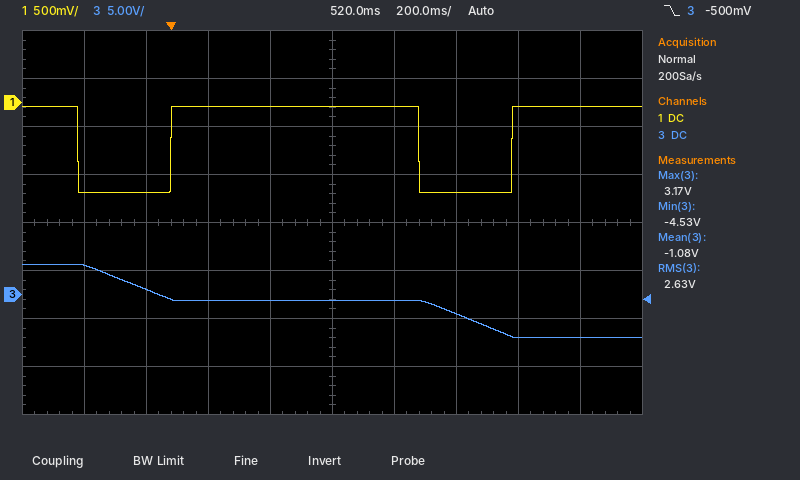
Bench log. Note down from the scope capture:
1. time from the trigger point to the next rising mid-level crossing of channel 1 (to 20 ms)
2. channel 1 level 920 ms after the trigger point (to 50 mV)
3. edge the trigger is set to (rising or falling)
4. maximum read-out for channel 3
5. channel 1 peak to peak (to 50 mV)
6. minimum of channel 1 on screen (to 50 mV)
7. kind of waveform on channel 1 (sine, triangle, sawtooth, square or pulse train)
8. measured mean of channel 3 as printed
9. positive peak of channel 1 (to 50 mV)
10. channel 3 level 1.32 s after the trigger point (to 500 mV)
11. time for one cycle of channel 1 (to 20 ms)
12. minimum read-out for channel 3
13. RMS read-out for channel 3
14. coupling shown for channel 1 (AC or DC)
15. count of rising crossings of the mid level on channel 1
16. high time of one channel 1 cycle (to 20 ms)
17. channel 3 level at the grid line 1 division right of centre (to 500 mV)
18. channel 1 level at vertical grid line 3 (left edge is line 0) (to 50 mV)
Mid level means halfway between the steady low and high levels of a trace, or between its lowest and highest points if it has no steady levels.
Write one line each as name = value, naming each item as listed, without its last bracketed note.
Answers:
time from the trigger point to the next rising mid-level crossing of channel 1 = 1.10 s
channel 1 level 920 ms after the trigger point = -950 mV
edge the trigger is set to = falling
maximum read-out for channel 3 = 3.17 V
channel 1 peak to peak = 900 mV
minimum of channel 1 on screen = -950 mV
kind of waveform on channel 1 = pulse train
measured mean of channel 3 as printed = -1.08 V
positive peak of channel 1 = -50 mV
channel 3 level 1.32 s after the trigger point = -4.5 V
time for one cycle of channel 1 = 1.10 s
minimum read-out for channel 3 = -4.53 V
RMS read-out for channel 3 = 2.63 V
coupling shown for channel 1 = DC
count of rising crossings of the mid level on channel 1 = 2
high time of one channel 1 cycle = 800 ms
channel 3 level at the grid line 1 division right of centre = -500 mV
channel 1 level at vertical grid line 3 (left edge is line 0) = -50 mV
